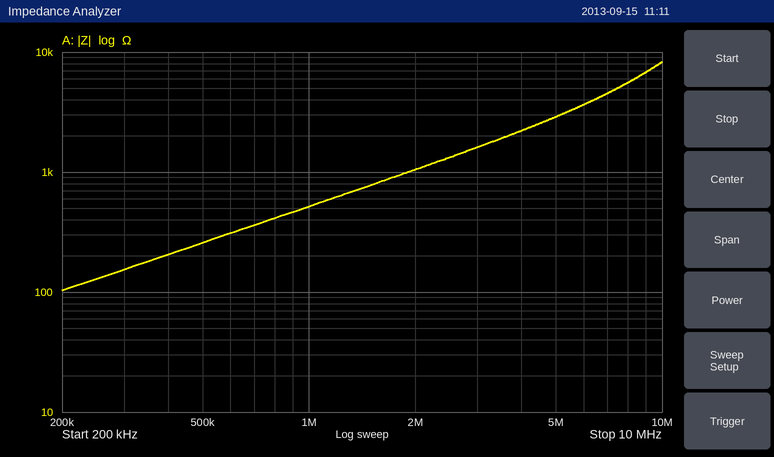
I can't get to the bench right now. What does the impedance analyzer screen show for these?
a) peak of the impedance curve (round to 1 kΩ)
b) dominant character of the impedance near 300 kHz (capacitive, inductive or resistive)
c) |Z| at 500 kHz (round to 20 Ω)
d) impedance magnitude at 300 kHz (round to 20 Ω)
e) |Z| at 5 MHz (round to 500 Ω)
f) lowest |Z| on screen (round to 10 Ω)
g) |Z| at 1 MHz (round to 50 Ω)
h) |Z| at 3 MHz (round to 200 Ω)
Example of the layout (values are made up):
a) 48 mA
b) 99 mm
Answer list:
a) 8 kΩ
b) inductive
c) 260 Ω
d) 160 Ω
e) 3.0 kΩ
f) 100 Ω
g) 500 Ω
h) 1.6 kΩ
